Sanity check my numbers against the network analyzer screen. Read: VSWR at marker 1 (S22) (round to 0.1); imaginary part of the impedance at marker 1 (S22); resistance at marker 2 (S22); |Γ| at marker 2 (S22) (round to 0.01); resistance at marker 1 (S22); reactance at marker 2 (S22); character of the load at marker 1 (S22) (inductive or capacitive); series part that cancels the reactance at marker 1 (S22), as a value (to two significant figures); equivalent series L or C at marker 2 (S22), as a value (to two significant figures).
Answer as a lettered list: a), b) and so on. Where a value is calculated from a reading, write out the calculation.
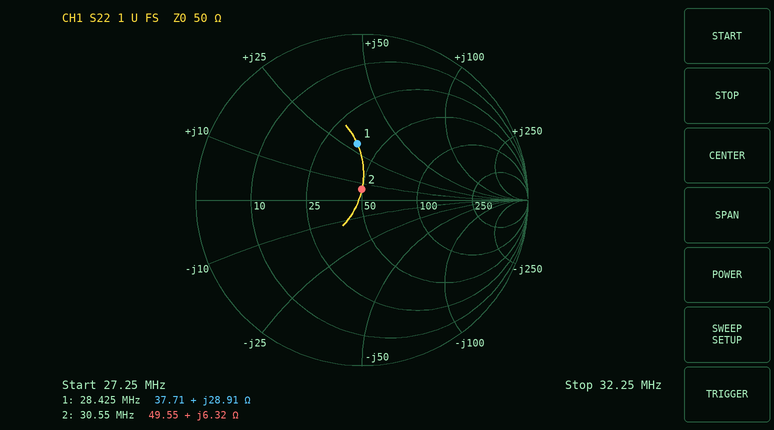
a) 2.0
b) +28.91 Ω
c) 49.55 Ω
d) 0.06
e) 37.71 Ω
f) +6.32 Ω
g) inductive
h) C = 1/(2π × 28.425 MHz × 28.91 Ω) ≈ 194 pF, so 190 pF to two significant figures
i) L = 6.32 Ω/(2π × 30.55 MHz) ≈ 33 nH
